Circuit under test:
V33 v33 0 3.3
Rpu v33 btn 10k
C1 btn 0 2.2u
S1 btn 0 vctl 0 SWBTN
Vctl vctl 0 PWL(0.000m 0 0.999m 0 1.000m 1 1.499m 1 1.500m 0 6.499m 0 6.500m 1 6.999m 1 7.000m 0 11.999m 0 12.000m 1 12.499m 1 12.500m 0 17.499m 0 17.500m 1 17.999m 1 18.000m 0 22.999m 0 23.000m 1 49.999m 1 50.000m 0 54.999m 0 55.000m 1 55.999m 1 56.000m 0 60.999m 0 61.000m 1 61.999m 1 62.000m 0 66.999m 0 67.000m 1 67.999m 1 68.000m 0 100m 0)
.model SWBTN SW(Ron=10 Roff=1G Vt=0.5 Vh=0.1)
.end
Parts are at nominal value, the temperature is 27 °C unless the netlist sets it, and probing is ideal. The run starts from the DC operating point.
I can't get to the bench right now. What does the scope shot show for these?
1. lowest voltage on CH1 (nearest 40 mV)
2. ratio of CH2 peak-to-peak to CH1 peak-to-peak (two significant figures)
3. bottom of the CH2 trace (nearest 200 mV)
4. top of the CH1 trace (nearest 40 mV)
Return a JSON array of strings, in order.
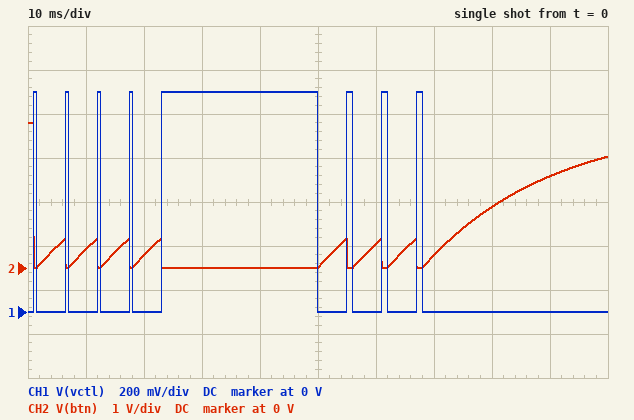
["0 V", "3.3", "0 V", "1.00 V"]
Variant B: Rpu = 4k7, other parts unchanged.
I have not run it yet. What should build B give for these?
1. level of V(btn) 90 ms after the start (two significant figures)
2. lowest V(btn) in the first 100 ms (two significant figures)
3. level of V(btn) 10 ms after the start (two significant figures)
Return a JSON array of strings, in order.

["2.9 V", "7.0 mV", "840 mV"]
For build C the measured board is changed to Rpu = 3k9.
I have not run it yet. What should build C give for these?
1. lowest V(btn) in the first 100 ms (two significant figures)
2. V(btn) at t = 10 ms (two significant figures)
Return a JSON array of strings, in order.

["8.4 mV", "980 mV"]
